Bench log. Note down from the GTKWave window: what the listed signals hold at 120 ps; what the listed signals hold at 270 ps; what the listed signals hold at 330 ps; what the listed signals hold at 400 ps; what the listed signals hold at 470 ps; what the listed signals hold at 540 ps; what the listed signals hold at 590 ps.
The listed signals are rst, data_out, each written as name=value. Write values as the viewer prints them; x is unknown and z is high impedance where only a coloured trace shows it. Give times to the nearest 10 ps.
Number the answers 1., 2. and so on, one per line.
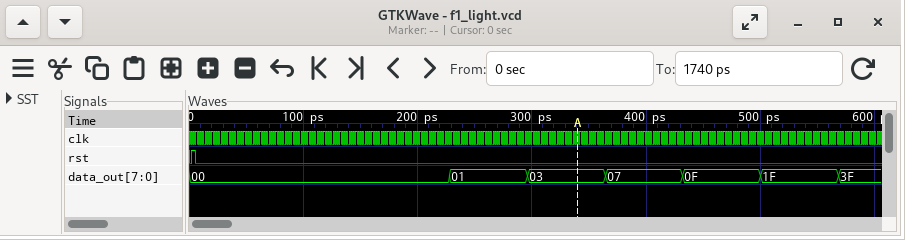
1. rst=0, data_out=00
2. rst=0, data_out=01
3. rst=0, data_out=03
4. rst=0, data_out=07
5. rst=0, data_out=0F
6. rst=0, data_out=1F
7. rst=0, data_out=3F
